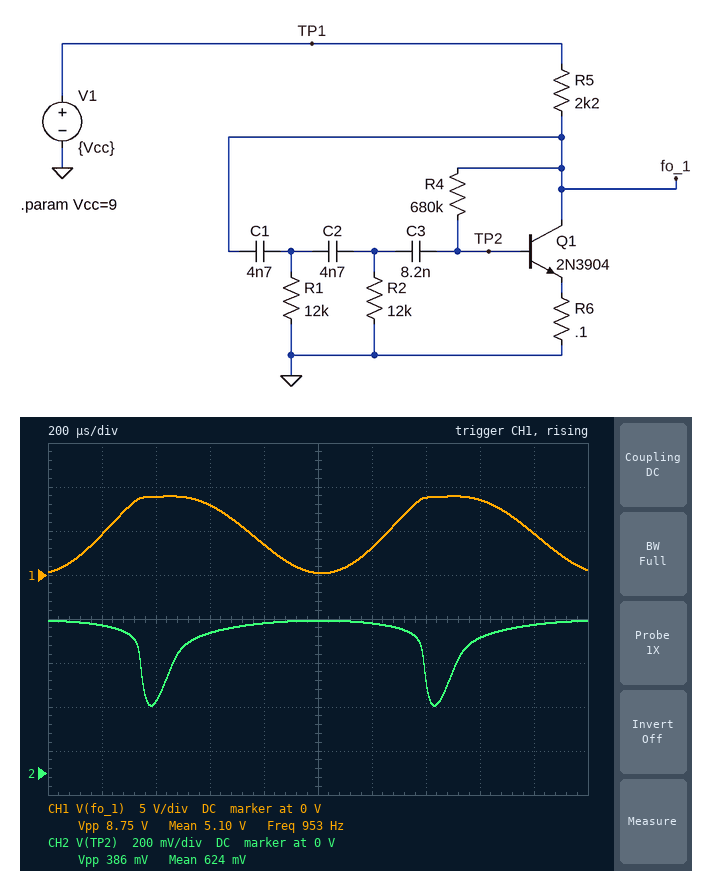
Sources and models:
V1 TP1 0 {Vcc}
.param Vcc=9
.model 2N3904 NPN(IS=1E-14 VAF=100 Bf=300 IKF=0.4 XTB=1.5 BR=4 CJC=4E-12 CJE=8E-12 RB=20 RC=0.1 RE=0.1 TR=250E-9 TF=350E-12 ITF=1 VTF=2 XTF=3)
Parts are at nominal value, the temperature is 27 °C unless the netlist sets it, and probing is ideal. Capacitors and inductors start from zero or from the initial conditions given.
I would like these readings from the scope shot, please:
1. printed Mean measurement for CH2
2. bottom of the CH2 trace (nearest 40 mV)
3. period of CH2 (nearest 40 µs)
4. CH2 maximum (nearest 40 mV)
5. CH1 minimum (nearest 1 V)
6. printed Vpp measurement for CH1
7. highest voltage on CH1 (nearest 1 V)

624 mV
320 mV
1.04 ms
680 mV
0 V
8.75 V
9 V
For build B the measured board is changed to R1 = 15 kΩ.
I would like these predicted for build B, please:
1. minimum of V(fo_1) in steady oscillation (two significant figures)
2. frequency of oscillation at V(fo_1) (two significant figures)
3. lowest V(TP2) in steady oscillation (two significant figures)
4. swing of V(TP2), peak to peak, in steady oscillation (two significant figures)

260 mV
890 Hz
340 mV
360 mV
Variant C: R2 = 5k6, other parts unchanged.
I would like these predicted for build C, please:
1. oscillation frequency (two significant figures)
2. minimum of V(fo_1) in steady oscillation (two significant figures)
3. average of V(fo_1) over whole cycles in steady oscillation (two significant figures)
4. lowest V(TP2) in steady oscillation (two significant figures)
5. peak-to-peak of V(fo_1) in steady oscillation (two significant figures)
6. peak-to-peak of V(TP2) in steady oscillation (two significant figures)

1.2 kHz
120 mV
5.0 V
330 mV
8.8 V
370 mV
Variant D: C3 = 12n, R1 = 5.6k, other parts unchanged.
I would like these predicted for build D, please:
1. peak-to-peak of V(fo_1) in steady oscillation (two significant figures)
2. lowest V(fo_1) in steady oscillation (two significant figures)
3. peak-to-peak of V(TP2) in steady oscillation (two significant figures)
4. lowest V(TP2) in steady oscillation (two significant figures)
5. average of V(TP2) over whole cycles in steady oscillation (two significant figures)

8.4 V
500 mV
260 mV
430 mV
640 mV
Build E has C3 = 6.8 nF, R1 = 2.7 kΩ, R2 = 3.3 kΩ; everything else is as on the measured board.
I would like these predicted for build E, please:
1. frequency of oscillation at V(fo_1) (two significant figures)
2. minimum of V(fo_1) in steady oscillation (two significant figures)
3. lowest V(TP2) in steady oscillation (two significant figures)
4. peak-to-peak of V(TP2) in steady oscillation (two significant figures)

2.4 kHz
100 mV
320 mV
370 mV
